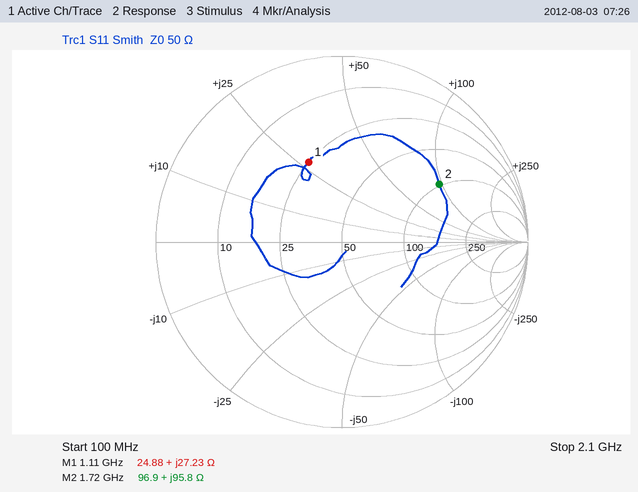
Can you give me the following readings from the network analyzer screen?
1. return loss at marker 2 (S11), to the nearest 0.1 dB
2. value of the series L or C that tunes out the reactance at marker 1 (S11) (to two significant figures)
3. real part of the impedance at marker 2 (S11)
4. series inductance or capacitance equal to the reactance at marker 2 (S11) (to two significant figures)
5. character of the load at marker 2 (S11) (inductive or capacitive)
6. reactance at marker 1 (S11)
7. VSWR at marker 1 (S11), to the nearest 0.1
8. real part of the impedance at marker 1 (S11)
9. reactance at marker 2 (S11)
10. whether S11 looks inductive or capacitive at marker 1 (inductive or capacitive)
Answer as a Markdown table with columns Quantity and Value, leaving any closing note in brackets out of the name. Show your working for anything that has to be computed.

| Quantity | Value |
|---|---|
| return loss at marker 2 (S11), to the nearest 0.1 dB | 4.3 dB |
| value of the series L or C that tunes out the reactance at marker 1 (S11) | C = 1/(2π × 1.11 GHz × 27.23 Ω) ≈ 5.3 pF |
| real part of the impedance at marker 2 | 96.9 Ω |
| series inductance or capacitance equal to the reactance at marker 2 (S11) | L = 95.8 Ω/(2π × 1.72 GHz) ≈ 8.9 nH |
| character of the load at marker 2 (S11) | inductive |
| reactance at marker 1 | +27.23 Ω |
| VSWR at marker 1 (S11), to the nearest 0.1 | 2.7 |
| real part of the impedance at marker 1 | 24.88 Ω |
| reactance at marker 2 | +95.8 Ω |
| whether S11 looks inductive or capacitive at marker 1 | inductive |
